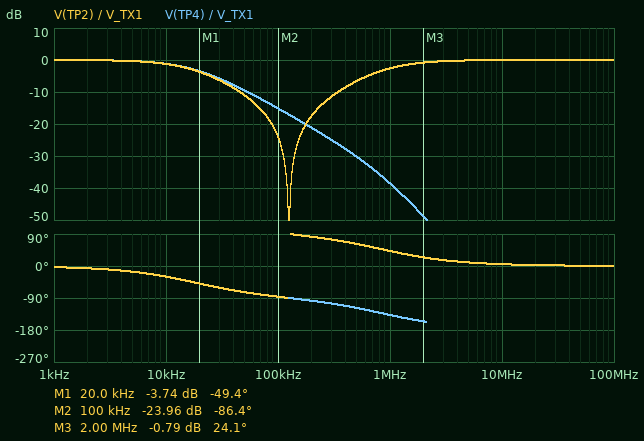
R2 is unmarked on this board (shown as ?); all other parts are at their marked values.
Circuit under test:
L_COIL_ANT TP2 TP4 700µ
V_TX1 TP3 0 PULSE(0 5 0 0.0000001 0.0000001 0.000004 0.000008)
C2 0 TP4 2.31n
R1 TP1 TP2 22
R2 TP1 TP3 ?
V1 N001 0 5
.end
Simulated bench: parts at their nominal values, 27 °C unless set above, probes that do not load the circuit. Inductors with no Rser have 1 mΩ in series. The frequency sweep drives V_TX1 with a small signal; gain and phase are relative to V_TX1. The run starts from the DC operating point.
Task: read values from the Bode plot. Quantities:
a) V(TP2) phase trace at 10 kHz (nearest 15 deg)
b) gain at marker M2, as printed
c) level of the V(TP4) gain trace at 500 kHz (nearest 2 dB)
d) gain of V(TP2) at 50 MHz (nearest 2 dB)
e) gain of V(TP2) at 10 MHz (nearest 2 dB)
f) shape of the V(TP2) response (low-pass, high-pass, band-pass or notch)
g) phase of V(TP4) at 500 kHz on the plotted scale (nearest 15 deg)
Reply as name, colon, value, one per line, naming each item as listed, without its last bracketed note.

V(TP2) phase trace at 10 kHz: -30 deg
gain at marker M2, as printed: -23.96 dB
level of the V(TP4) gain trace at 500 kHz: -30 dB
gain of V(TP2) at 50 MHz: 0 dB
gain of V(TP2) at 10 MHz: 0 dB
shape of the V(TP2) response: notch
phase of V(TP4) at 500 kHz on the plotted scale: -120 deg
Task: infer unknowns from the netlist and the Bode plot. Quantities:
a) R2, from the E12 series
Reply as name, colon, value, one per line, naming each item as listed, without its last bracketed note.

R2, from the E12 series: 3.9 kΩ
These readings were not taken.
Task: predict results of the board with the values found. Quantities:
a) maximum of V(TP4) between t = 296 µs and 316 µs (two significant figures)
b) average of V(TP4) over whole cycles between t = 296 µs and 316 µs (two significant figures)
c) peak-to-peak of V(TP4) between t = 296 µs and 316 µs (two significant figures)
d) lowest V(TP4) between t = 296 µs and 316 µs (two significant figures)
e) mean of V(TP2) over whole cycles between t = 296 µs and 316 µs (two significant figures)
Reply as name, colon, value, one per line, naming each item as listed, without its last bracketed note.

maximum of V(TP4) between t = 296 µs and 316 µs: 3.1 V
average of V(TP4) over whole cycles between t = 296 µs and 316 µs: 2.6 V
peak-to-peak of V(TP4) between t = 296 µs and 316 µs: 1.0 V
lowest V(TP4) between t = 296 µs and 316 µs: 2.0 V
mean of V(TP2) over whole cycles between t = 296 µs and 316 µs: 2.6 V
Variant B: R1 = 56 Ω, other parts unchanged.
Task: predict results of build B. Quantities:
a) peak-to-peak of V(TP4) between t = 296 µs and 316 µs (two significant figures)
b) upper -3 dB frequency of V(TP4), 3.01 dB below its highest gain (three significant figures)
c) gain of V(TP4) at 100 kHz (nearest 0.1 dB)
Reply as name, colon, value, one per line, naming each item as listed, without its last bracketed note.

peak-to-peak of V(TP4) between t = 296 µs and 316 µs: 1.0 V
upper -3 dB frequency of V(TP4), 3.01 dB below its highest gain: 17.8 kHz
gain of V(TP4) at 100 kHz: -15.2 dB
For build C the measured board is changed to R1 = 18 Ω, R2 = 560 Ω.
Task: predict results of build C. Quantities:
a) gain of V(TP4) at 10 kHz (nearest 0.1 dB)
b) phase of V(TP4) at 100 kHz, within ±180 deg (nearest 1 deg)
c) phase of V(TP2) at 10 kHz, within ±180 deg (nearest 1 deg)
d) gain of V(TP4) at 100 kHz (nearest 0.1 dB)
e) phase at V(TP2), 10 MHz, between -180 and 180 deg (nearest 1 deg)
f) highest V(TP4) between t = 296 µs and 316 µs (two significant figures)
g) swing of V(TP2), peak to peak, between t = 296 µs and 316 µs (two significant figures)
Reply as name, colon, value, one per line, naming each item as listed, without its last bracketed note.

gain of V(TP4) at 10 kHz: 0 dB
phase of V(TP4) at 100 kHz, within ±180 deg: -67 deg
phase of V(TP2) at 10 kHz, within ±180 deg: -5 deg
gain of V(TP4) at 100 kHz: 0.8 dB
phase at V(TP2), 10 MHz, between -180 and 180 deg: 1 deg
highest V(TP4) between t = 296 µs and 316 µs: 5.7 V
swing of V(TP2), peak to peak, between t = 296 µs and 316 µs: 6.0 V
